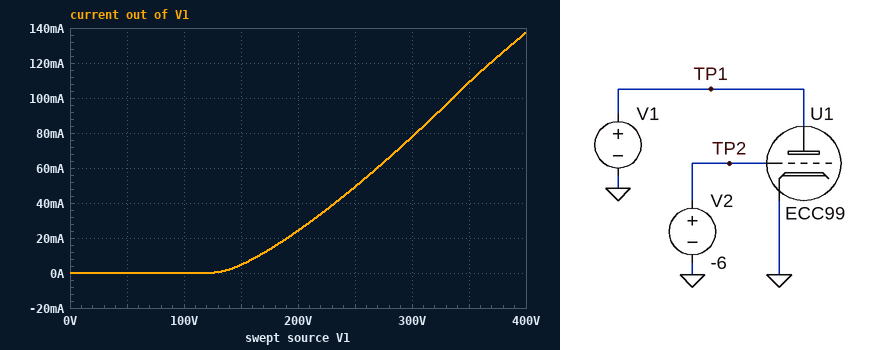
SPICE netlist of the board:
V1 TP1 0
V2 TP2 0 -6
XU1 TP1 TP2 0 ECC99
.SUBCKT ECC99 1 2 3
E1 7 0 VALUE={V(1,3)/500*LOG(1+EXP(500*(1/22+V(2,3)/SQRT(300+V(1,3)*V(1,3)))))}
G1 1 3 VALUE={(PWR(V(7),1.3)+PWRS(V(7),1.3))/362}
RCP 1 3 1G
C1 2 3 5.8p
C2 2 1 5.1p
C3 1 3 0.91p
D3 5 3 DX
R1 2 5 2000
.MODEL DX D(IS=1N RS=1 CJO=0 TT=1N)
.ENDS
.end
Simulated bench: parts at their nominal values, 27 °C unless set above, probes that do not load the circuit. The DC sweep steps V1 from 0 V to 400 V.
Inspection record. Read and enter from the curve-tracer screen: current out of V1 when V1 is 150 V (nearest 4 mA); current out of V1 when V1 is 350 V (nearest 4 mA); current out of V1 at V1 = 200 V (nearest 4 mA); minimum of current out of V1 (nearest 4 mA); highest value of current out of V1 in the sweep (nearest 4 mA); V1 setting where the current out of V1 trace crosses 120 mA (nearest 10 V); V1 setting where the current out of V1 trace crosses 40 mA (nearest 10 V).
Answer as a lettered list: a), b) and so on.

a) 4 mA
b) 108 mA
c) 24 mA
d) 0 A
e) 136 mA
f) 370 V
g) 230 V
